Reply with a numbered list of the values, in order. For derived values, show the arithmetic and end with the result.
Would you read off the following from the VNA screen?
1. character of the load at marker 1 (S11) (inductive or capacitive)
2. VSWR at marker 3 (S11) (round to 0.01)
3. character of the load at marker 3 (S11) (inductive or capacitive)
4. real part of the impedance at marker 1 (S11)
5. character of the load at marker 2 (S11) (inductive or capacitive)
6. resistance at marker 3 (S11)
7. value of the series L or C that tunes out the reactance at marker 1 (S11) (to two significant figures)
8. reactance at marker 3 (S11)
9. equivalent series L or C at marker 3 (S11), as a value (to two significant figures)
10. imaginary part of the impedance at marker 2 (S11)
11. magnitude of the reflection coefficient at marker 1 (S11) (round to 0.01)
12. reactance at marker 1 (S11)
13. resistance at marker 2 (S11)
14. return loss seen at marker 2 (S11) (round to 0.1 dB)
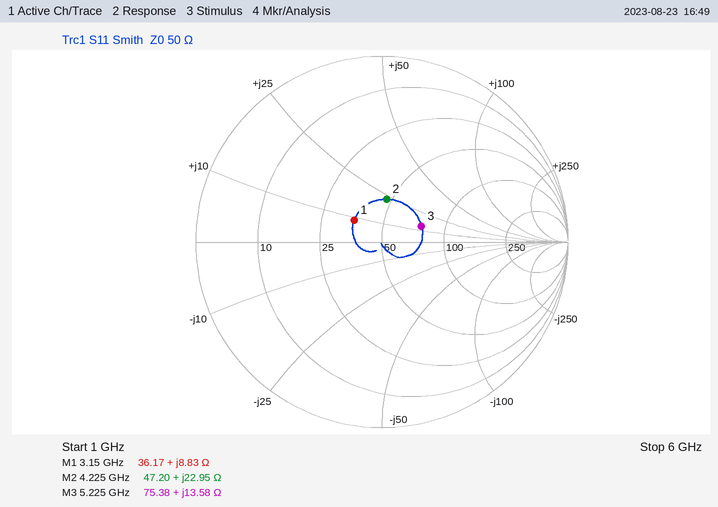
1. inductive
2. 1.59
3. inductive
4. 36.17 Ω
5. inductive
6. 75.38 Ω
7. C = 1/(2π × 3.15 GHz × 8.83 Ω) ≈ 5.7 pF
8. +13.58 Ω
9. L = 13.58 Ω/(2π × 5.225 GHz) ≈ 414 pH, so 410 pH to two significant figures
10. +22.95 Ω
11. 0.19
12. +8.83 Ω
13. 47.20 Ω
14. 12.7 dB
